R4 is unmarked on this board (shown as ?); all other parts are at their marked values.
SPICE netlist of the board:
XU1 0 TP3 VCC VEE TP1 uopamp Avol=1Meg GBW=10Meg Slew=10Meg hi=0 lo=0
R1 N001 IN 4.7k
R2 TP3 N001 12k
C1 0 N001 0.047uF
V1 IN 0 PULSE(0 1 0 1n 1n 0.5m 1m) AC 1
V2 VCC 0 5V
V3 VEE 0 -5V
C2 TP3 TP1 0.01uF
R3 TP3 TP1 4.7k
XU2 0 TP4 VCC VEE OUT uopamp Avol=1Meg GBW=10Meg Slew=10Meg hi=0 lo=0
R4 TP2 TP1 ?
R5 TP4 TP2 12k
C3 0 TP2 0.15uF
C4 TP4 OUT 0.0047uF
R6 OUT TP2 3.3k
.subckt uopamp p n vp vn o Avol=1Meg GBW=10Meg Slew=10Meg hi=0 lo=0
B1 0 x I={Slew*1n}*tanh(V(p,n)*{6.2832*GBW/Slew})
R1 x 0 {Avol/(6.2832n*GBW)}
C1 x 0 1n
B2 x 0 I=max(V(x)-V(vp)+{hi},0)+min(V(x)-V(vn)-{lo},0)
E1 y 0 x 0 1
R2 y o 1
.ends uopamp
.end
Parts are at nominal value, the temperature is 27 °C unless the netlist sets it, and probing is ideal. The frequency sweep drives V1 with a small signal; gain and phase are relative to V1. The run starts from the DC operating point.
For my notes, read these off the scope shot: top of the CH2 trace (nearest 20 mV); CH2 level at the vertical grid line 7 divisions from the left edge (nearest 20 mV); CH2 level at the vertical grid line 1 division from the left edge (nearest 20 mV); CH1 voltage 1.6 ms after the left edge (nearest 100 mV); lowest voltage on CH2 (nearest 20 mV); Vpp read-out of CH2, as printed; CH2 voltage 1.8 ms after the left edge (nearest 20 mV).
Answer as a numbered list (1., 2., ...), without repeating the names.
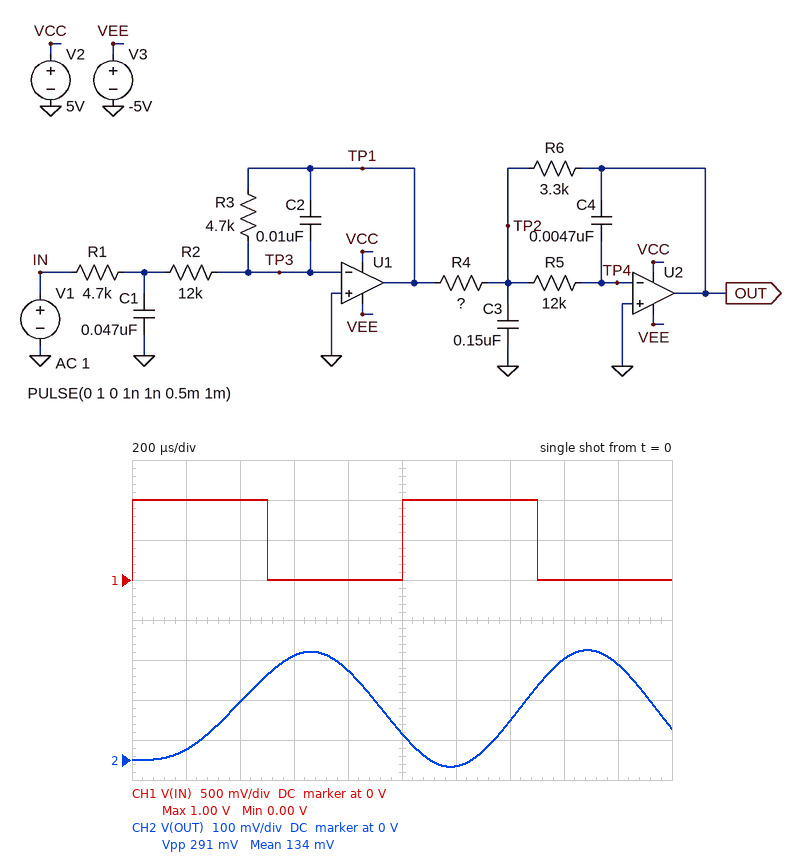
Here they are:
1. 280 mV
2. 100 mV
3. 20 mV
4. 0 V
5. -20 mV
6. 291 mV
7. 240 mV
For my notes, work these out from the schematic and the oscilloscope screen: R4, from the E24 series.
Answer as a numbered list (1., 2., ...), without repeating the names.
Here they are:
1. 3.6 kΩ
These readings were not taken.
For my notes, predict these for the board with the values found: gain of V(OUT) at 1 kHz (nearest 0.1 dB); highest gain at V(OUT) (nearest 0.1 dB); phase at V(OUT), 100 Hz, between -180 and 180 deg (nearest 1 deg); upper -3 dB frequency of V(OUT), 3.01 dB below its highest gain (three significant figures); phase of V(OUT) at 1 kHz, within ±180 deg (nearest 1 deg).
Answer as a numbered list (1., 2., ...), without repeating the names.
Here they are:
1. -13.0 dB
2. -10.7 dB
3. -12 deg
4. 1.04 kHz
5. -159 deg
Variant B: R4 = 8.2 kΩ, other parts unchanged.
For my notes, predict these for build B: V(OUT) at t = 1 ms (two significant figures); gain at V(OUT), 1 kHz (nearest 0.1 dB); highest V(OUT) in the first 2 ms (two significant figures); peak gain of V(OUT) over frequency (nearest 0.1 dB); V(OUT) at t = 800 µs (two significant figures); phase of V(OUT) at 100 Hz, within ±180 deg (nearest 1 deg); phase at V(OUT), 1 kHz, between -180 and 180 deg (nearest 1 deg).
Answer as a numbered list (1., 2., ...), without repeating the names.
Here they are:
1. 20 mV
2. -17.9 dB
3. 140 mV
4. -16.2 dB
5. 100 mV
6. -11 deg
7. -161 deg
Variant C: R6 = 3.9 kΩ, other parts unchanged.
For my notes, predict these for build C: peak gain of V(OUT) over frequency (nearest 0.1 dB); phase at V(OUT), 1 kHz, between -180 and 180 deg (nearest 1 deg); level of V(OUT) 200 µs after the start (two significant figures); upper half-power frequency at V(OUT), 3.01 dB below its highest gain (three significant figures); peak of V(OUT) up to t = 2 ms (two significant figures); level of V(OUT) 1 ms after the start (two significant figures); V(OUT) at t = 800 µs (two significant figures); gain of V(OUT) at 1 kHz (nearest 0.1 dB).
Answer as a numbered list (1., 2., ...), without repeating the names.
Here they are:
1. -9.1 dB
2. -171 deg
3. 26 mV
4. 964 Hz
5. 310 mV
6. 110 mV
7. 280 mV
8. -12.8 dB
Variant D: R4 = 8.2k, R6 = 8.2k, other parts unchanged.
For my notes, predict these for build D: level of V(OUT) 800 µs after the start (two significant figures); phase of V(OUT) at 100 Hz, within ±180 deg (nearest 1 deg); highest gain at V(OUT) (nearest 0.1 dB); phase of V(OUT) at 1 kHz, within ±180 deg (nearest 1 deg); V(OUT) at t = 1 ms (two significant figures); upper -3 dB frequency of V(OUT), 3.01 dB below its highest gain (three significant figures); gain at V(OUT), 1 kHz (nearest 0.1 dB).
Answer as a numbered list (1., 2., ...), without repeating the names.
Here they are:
1. 270 mV
2. -13 deg
3. -7.1 dB
4. 147 deg
5. 220 mV
6. 690 Hz
7. -20.3 dB
